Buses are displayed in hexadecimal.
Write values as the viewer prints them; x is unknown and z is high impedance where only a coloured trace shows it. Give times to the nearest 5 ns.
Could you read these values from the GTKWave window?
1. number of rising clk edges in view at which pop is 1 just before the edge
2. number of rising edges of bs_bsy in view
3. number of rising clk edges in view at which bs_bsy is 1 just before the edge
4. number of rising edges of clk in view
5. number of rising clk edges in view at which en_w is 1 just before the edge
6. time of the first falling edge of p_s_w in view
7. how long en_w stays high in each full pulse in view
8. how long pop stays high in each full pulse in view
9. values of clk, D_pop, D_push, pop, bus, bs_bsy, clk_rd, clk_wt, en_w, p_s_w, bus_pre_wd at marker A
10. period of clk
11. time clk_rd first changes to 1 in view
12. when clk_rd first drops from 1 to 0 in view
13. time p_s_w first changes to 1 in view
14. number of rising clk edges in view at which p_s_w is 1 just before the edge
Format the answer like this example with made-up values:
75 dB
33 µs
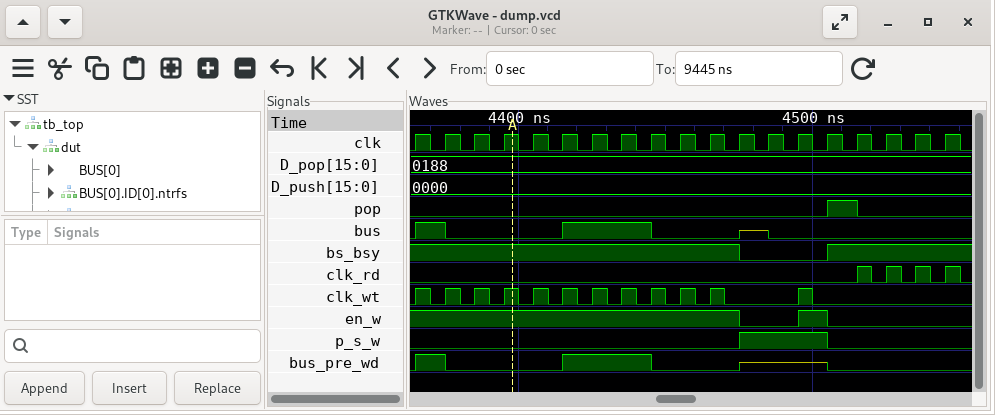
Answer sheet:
1
1
16
19
13
4505 ns
10 ns
10 ns
clk=1, D_pop=0188, D_push=0000, pop=0, bus=0, bs_bsy=1, clk_rd=0, clk_wt=1, en_w=1, p_s_w=0, bus_pre_wd=0
10 ns
4515 ns
4520 ns
4475 ns
3
